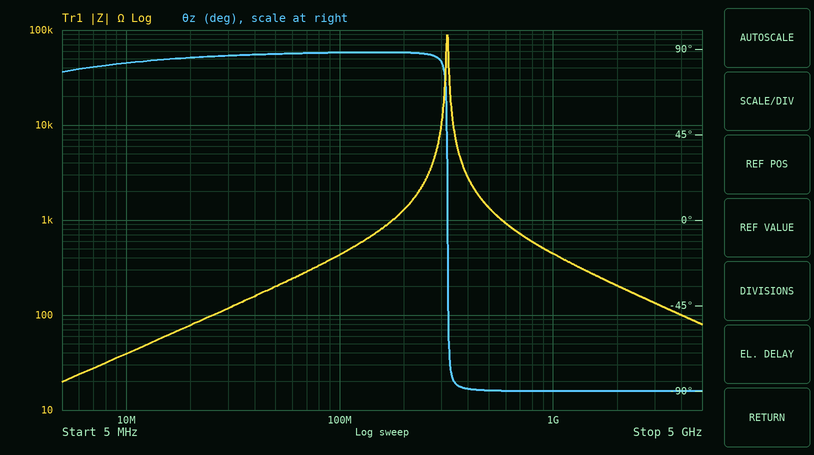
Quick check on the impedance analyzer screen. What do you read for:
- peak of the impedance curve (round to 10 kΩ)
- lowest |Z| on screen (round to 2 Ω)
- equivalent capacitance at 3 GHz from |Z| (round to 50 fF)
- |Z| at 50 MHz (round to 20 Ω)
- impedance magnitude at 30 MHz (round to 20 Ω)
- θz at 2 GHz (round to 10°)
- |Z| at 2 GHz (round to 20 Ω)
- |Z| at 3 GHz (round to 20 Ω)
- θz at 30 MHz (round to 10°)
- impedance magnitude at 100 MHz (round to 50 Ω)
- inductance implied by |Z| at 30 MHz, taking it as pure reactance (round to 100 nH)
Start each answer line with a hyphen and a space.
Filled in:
- 90 kΩ
- 20 Ω
- 400 fF
- 200 Ω
- 120 Ω
- -90°
- 200 Ω
- 140 Ω
- 90°
- 450 Ω
- 600 nH
